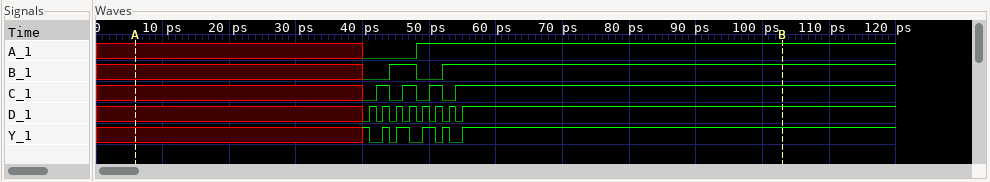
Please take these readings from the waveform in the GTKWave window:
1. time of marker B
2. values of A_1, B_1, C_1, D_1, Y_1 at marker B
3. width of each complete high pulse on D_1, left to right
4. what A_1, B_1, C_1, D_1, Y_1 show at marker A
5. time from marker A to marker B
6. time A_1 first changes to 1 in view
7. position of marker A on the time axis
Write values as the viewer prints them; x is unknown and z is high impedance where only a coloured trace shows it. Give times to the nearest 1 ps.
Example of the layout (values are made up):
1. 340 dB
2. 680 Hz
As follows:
1. 103 ps
2. A_1=1, B_1=1, C_1=1, D_1=1, Y_1=1
3. 1 ps, 1 ps, 1 ps, 1 ps, 1 ps, 1 ps, 1 ps
4. A_1=x, B_1=x, C_1=x, D_1=x, Y_1=x
5. 97 ps
6. 48 ps
7. 6 ps
